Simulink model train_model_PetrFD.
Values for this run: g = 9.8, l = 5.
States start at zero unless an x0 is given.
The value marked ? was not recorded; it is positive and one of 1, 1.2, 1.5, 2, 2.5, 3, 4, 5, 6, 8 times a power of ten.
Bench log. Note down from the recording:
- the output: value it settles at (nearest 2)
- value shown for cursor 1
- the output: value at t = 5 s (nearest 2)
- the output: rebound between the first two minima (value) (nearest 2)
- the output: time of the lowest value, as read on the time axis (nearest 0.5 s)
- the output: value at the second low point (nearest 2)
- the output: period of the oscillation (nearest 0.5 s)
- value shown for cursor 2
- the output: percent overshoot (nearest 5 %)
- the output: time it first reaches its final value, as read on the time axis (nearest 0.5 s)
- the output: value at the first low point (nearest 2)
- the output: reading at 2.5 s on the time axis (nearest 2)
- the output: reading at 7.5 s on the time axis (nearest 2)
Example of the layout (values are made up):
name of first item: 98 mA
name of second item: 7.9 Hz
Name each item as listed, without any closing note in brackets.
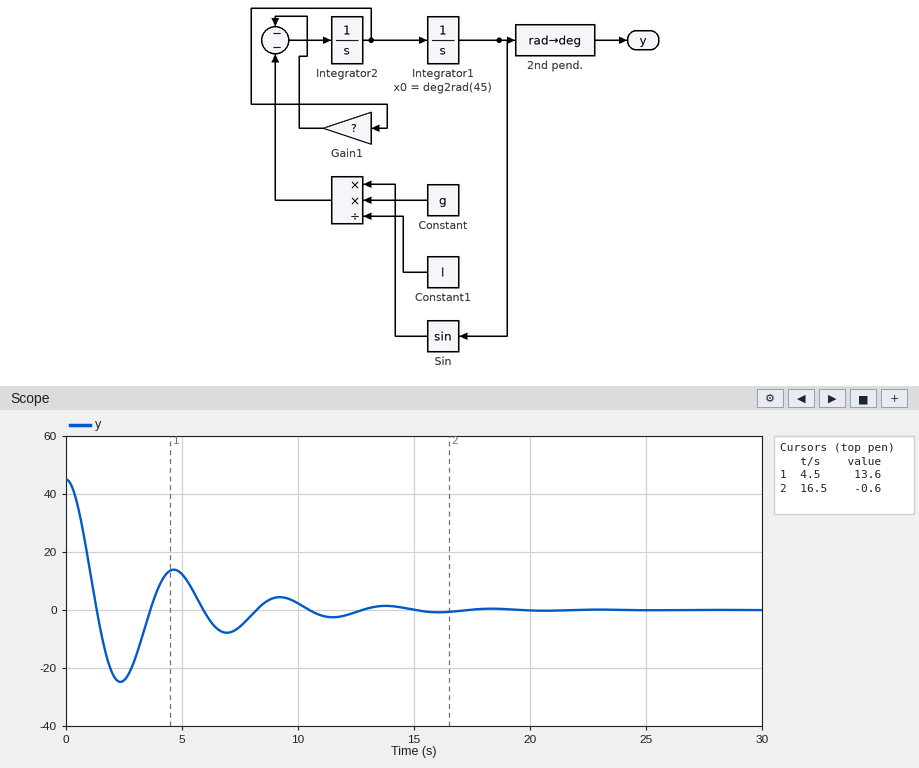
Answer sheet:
the output: value it settles at: 0
value shown for cursor 1: 13.6
the output: value at t = 5 s: 12
the output: rebound between the first two minima (value): 14
the output: time of the lowest value, as read on the time axis: 2.5 s
the output: value at the second low point: -8
the output: period of the oscillation: 4.5 s
value shown for cursor 2: -0.6
the output: percent overshoot: 55 %
the output: time it first reaches its final value, as read on the time axis: 1.5 s
the output: value at the first low point: -24
the output: reading at 2.5 s on the time axis: -24
the output: reading at 7.5 s on the time axis: -6
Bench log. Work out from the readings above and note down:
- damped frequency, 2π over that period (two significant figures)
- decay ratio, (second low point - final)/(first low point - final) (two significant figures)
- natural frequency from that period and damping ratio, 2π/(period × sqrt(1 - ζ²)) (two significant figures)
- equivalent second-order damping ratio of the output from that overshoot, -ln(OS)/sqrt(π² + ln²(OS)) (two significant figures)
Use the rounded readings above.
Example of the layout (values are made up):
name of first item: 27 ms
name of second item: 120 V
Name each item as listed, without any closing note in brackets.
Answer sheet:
damped frequency, 2π over that period: 1.4 rad/s
decay ratio, (second low point - final)/(first low point - final): 0.33
natural frequency from that period and damping ratio, 2π/(period × sqrt(1 - ζ²)): 1.4 rad/s
equivalent second-order damping ratio of the output from that overshoot, -ln(OS)/sqrt(π² + ln²(OS)): 0.19
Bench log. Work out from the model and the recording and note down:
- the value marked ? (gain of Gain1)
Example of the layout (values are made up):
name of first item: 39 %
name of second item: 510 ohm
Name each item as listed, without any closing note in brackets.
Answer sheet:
the value marked ?: 0.5
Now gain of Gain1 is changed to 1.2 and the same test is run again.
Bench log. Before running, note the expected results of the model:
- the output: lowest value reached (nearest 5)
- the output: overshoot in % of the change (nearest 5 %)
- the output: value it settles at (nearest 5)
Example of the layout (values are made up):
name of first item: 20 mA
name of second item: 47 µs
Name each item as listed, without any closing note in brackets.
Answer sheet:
the output: lowest value reached: -10
the output: overshoot in % of the change: 20 %
the output: value it settles at: 0
